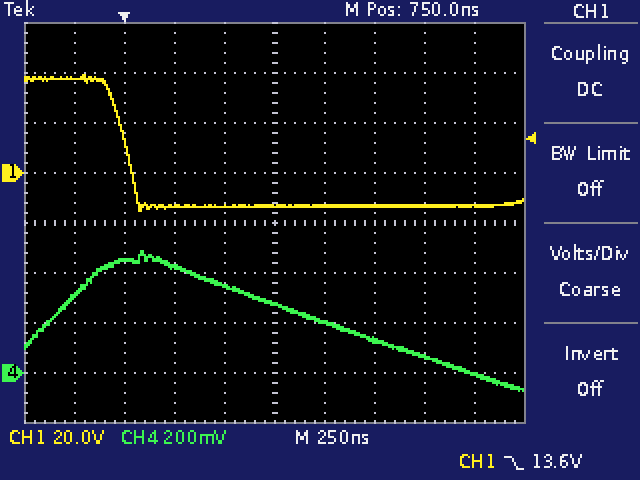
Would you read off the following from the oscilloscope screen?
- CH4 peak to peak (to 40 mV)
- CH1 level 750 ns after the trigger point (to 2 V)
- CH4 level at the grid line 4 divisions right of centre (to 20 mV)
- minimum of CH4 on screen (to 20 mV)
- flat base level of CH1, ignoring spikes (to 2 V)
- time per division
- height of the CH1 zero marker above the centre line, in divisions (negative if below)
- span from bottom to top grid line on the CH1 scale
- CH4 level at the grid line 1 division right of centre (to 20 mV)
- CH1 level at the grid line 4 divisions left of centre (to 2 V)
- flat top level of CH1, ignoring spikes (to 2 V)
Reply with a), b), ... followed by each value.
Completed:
a) 560 mV
b) -14 V
c) 0 mV
d) -80 mV
e) -14 V
f) 250 ns
g) +1.0 div
h) 160 V
i) 200 mV
j) 38 V
k) 38 V
